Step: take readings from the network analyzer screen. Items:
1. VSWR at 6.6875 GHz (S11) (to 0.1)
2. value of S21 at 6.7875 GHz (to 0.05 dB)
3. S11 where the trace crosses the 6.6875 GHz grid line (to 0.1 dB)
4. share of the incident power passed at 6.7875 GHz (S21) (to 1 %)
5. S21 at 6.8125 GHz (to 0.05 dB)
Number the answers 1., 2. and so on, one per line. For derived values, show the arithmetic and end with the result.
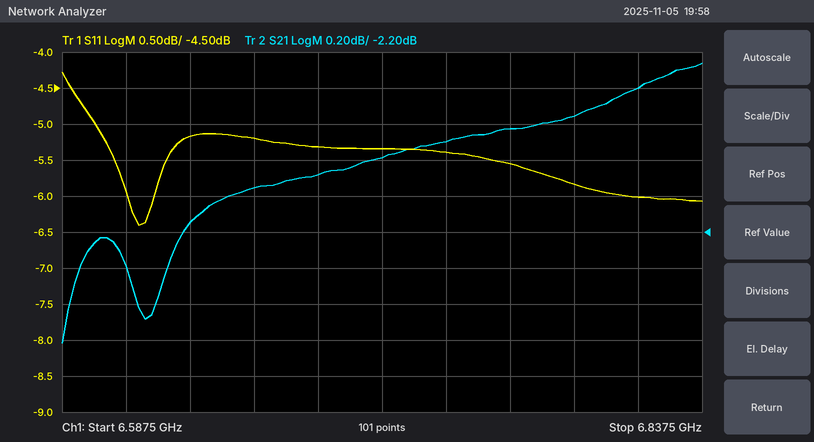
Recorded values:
1. |Γ| = 10^(-5.3/20) = 0.5433; VSWR = (1 + 0.5433)/(1 − 0.5433) ≈ 3.4
2. -1.55 dB
3. -5.3 dB
4. 10^(-1.55/10) ≈ 70 %
5. -1.40 dB
